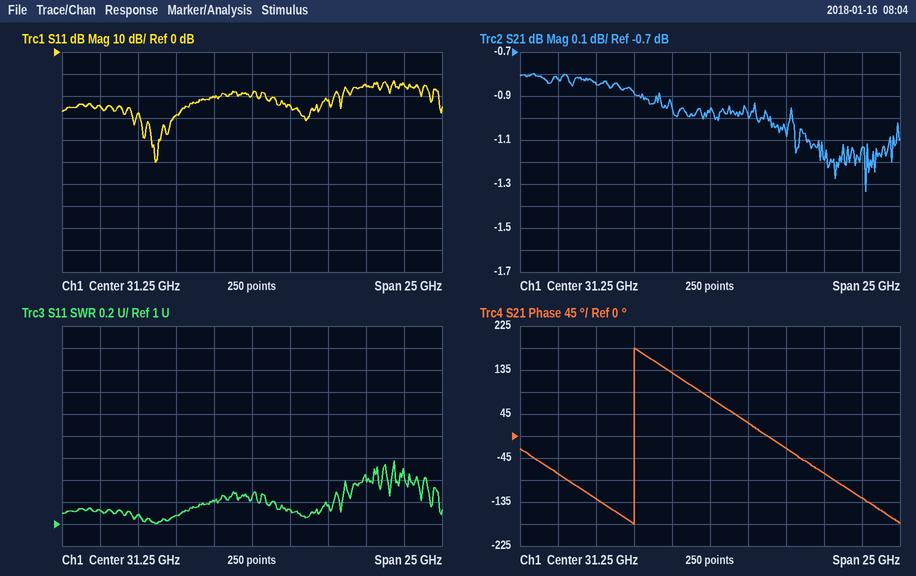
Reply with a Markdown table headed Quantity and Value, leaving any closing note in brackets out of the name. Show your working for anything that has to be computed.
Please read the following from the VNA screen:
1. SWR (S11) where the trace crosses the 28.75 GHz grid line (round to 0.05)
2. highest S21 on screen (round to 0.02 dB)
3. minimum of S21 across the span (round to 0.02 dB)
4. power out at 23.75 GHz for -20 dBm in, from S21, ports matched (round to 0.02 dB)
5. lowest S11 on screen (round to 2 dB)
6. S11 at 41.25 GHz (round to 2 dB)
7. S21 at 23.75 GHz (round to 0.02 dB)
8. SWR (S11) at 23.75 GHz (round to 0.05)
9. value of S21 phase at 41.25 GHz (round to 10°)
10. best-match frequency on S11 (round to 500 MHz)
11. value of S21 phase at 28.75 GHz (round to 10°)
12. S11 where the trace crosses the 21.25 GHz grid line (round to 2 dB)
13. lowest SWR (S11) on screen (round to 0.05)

| Quantity | Value |
|---|---|
| SWR (S11) where the trace crosses the 28.75 GHz grid line | 1.20 |
| highest S21 on screen | -0.80 dB |
| minimum of S21 across the span | -1.34 dB |
| power out at 23.75 GHz for -20 dBm in, from S21, ports matched | -20 dBm + (-0.84 dB) = -20.84 dBm |
| lowest S11 on screen | -50 dB |
| S11 at 41.25 GHz | -14 dB |
| S21 at 23.75 GHz | -0.84 dB |
| SWR (S11) at 23.75 GHz | 1.10 |
| value of S21 phase at 41.25 GHz | -130° |
| best-match frequency on S11 | 25.0 GHz |
| value of S21 phase at 28.75 GHz | 130° |
| S11 where the trace crosses the 21.25 GHz grid line | -24 dB |
| lowest SWR (S11) on screen | 1.00 |
